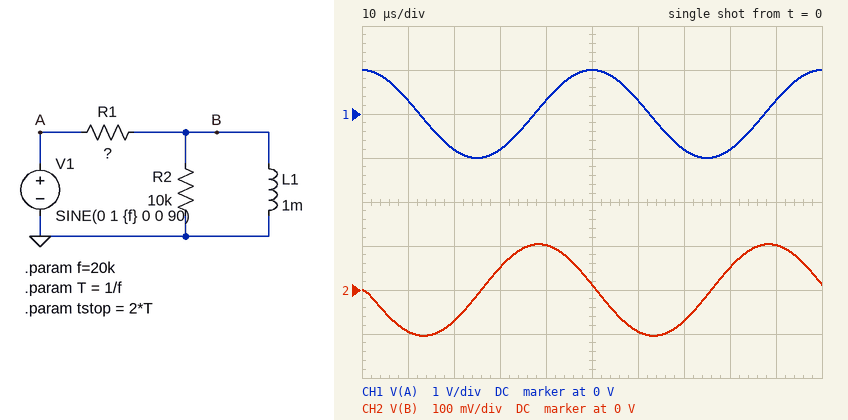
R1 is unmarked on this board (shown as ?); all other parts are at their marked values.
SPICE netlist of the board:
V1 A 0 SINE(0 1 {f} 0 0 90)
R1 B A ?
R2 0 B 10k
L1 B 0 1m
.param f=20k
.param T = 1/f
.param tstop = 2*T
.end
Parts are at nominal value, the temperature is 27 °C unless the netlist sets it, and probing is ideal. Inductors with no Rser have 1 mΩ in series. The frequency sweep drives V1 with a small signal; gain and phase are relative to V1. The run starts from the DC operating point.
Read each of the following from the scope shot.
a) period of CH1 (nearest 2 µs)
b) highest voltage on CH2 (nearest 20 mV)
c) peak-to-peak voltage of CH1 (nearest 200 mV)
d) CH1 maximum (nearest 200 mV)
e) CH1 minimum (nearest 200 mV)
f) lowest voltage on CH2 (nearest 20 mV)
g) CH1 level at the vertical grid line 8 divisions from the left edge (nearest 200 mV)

50 µs
100 mV
2.0 V
1.0 V
-1.0 V
-100 mV
-800 mV
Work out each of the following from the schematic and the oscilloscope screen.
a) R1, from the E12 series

1.2 kΩ
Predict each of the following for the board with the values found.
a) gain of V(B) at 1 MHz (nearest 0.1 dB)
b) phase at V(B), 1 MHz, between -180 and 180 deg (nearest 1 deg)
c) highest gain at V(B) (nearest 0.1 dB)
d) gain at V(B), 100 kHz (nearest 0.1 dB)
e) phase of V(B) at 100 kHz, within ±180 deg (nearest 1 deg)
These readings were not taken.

-1.1 dB
10 deg
-1.0 dB
-6.9 dB
60 deg
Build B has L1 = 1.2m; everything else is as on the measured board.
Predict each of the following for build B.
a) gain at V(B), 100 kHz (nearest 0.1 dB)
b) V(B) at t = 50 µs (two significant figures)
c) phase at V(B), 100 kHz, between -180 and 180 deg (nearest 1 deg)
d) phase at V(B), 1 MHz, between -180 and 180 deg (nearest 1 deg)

-5.8 dB
17 mV
55 deg
8 deg
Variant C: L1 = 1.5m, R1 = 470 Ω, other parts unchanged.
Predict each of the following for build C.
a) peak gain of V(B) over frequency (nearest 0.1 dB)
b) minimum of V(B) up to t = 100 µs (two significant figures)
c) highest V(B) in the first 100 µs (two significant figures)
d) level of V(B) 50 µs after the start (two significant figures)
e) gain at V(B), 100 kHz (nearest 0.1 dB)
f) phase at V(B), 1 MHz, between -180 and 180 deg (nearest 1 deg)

-0.4 dB
-370 mV
370 mV
140 mV
-1.3 dB
3 deg
